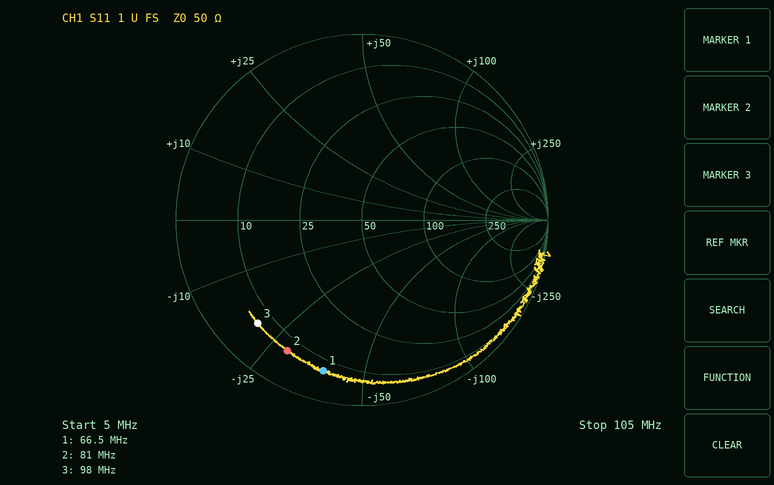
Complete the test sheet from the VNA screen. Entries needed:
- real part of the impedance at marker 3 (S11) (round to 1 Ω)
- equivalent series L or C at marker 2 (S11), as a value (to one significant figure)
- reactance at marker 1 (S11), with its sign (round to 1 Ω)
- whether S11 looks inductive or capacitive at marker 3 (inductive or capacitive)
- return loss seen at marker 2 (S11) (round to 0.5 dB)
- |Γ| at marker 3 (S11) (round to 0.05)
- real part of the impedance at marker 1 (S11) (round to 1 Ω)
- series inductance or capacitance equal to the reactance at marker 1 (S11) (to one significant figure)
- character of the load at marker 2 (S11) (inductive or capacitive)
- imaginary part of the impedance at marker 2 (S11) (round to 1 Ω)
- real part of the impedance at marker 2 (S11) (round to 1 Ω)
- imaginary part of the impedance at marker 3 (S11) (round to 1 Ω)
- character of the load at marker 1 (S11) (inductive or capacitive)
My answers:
7 Ω
70 pF
-38 Ω
capacitive
2.0 dB
0.80
7 Ω
60 pF
capacitive
-29 Ω
7 Ω
-20 Ω
capacitive
